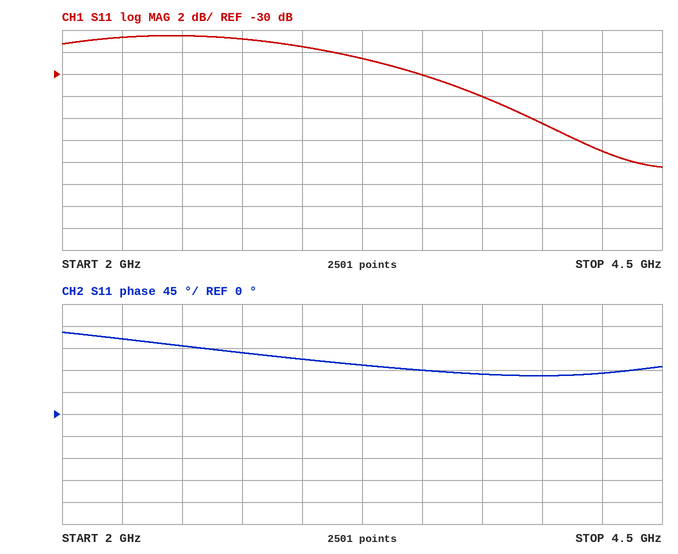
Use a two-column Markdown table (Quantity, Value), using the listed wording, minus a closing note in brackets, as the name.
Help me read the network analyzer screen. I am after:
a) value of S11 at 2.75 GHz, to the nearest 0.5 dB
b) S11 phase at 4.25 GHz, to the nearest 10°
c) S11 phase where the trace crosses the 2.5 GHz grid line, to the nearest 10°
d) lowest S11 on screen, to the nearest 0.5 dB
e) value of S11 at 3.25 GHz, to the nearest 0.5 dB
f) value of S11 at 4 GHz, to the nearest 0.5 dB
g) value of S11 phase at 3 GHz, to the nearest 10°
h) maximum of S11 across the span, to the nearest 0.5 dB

| Quantity | Value |
|---|---|
| value of S11 at 2.75 GHz, to the nearest 0.5 dB | -27.0 dB |
| S11 phase at 4.25 GHz, to the nearest 10° | 80° |
| S11 phase where the trace crosses the 2.5 GHz grid line, to the nearest 10° | 140° |
| lowest S11 on screen, to the nearest 0.5 dB | -38.5 dB |
| value of S11 at 3.25 GHz, to the nearest 0.5 dB | -28.5 dB |
| value of S11 at 4 GHz, to the nearest 0.5 dB | -34.5 dB |
| value of S11 phase at 3 GHz, to the nearest 10° | 110° |
| maximum of S11 across the span, to the nearest 0.5 dB | -26.5 dB |
